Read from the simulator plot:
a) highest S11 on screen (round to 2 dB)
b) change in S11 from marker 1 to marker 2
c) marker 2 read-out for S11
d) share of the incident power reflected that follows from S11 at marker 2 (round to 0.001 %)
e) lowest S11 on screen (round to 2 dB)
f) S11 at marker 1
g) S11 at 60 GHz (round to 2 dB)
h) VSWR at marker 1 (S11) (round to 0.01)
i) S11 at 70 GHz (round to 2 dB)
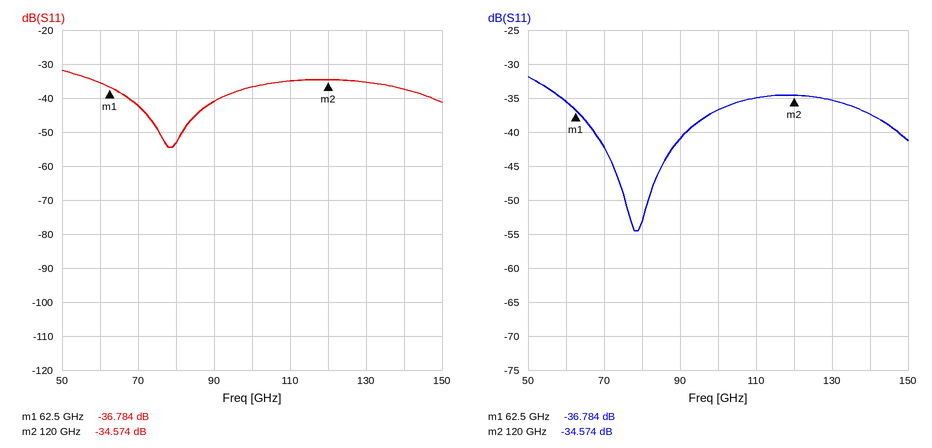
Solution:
-32 dB
2.210 dB
-34.574 dB
0.035 %
-54 dB
-36.784 dB
-36 dB
1.03
-42 dB
